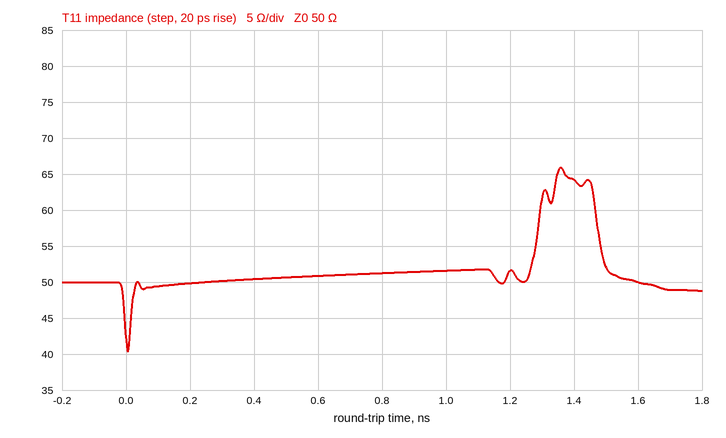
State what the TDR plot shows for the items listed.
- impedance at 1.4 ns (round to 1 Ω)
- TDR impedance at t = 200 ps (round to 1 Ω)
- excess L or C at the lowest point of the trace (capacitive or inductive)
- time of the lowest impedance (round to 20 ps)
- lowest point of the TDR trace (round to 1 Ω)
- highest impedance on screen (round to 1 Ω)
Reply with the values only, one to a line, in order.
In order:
64 Ω
50 Ω
capacitive
0 ps
40 Ω
66 Ω
